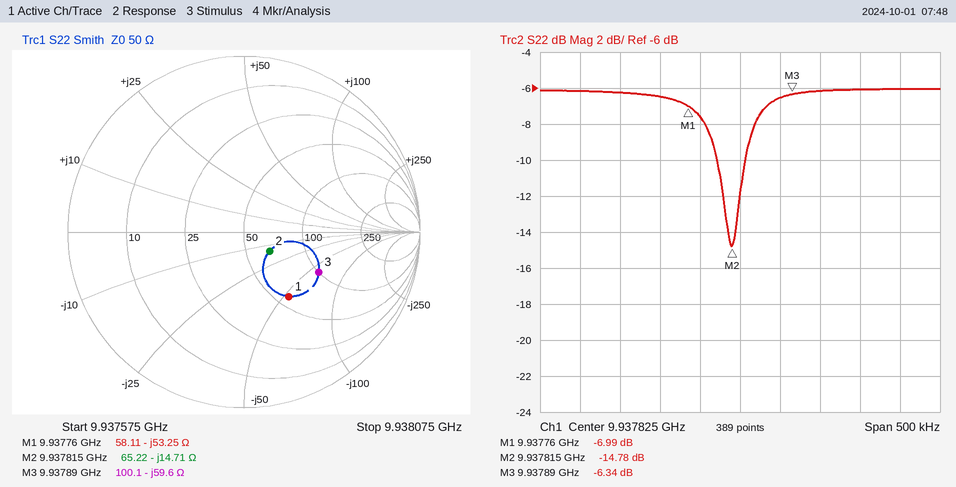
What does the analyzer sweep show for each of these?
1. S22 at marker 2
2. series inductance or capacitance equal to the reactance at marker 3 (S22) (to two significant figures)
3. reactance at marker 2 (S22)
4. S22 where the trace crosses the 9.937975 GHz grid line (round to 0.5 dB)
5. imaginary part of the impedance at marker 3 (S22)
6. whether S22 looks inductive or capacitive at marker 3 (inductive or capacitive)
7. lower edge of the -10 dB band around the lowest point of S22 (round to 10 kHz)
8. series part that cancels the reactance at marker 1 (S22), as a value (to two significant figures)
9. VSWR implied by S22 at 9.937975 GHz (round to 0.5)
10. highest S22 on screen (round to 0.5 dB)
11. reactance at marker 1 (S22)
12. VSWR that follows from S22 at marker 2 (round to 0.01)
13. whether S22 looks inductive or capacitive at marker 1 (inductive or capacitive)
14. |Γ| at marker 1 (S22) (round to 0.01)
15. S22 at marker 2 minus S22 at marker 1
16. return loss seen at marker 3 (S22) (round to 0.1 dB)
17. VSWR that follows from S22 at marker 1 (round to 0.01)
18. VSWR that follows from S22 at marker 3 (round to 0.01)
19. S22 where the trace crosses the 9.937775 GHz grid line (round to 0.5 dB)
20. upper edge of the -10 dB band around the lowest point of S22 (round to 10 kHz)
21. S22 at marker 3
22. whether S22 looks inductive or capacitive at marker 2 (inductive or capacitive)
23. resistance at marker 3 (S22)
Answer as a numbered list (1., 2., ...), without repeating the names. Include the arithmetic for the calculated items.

1. -14.78 dB
2. C = 1/(2π × 9.93789 GHz × 59.6 Ω) ≈ 269 fF, so 270 fF to two significant figures
3. -14.71 Ω
4. -6.0 dB
5. -59.6 Ω
6. capacitive
7. 9.93780 GHz
8. L = 53.25 Ω/(2π × 9.93776 GHz) ≈ 853 pH, so 850 pH to two significant figures
9. |Γ| = 10^(-6/20) = 0.5012; VSWR = (1 + 0.5012)/(1 − 0.5012) ≈ 3.0
10. -6.0 dB
11. -53.25 Ω
12. (1 + 0.1824)/(1 − 0.1824) ≈ 1.45
13. capacitive
14. 0.45
15. -14.78 − (-6.99) = -7.79 dB
16. 6.3 dB
17. (1 + 0.4472)/(1 − 0.4472) ≈ 2.62
18. (1 + 0.4819)/(1 − 0.4819) ≈ 2.86
19. -7.5 dB
20. 9.93783 GHz
21. -6.34 dB
22. capacitive
23. 100.1 Ω
